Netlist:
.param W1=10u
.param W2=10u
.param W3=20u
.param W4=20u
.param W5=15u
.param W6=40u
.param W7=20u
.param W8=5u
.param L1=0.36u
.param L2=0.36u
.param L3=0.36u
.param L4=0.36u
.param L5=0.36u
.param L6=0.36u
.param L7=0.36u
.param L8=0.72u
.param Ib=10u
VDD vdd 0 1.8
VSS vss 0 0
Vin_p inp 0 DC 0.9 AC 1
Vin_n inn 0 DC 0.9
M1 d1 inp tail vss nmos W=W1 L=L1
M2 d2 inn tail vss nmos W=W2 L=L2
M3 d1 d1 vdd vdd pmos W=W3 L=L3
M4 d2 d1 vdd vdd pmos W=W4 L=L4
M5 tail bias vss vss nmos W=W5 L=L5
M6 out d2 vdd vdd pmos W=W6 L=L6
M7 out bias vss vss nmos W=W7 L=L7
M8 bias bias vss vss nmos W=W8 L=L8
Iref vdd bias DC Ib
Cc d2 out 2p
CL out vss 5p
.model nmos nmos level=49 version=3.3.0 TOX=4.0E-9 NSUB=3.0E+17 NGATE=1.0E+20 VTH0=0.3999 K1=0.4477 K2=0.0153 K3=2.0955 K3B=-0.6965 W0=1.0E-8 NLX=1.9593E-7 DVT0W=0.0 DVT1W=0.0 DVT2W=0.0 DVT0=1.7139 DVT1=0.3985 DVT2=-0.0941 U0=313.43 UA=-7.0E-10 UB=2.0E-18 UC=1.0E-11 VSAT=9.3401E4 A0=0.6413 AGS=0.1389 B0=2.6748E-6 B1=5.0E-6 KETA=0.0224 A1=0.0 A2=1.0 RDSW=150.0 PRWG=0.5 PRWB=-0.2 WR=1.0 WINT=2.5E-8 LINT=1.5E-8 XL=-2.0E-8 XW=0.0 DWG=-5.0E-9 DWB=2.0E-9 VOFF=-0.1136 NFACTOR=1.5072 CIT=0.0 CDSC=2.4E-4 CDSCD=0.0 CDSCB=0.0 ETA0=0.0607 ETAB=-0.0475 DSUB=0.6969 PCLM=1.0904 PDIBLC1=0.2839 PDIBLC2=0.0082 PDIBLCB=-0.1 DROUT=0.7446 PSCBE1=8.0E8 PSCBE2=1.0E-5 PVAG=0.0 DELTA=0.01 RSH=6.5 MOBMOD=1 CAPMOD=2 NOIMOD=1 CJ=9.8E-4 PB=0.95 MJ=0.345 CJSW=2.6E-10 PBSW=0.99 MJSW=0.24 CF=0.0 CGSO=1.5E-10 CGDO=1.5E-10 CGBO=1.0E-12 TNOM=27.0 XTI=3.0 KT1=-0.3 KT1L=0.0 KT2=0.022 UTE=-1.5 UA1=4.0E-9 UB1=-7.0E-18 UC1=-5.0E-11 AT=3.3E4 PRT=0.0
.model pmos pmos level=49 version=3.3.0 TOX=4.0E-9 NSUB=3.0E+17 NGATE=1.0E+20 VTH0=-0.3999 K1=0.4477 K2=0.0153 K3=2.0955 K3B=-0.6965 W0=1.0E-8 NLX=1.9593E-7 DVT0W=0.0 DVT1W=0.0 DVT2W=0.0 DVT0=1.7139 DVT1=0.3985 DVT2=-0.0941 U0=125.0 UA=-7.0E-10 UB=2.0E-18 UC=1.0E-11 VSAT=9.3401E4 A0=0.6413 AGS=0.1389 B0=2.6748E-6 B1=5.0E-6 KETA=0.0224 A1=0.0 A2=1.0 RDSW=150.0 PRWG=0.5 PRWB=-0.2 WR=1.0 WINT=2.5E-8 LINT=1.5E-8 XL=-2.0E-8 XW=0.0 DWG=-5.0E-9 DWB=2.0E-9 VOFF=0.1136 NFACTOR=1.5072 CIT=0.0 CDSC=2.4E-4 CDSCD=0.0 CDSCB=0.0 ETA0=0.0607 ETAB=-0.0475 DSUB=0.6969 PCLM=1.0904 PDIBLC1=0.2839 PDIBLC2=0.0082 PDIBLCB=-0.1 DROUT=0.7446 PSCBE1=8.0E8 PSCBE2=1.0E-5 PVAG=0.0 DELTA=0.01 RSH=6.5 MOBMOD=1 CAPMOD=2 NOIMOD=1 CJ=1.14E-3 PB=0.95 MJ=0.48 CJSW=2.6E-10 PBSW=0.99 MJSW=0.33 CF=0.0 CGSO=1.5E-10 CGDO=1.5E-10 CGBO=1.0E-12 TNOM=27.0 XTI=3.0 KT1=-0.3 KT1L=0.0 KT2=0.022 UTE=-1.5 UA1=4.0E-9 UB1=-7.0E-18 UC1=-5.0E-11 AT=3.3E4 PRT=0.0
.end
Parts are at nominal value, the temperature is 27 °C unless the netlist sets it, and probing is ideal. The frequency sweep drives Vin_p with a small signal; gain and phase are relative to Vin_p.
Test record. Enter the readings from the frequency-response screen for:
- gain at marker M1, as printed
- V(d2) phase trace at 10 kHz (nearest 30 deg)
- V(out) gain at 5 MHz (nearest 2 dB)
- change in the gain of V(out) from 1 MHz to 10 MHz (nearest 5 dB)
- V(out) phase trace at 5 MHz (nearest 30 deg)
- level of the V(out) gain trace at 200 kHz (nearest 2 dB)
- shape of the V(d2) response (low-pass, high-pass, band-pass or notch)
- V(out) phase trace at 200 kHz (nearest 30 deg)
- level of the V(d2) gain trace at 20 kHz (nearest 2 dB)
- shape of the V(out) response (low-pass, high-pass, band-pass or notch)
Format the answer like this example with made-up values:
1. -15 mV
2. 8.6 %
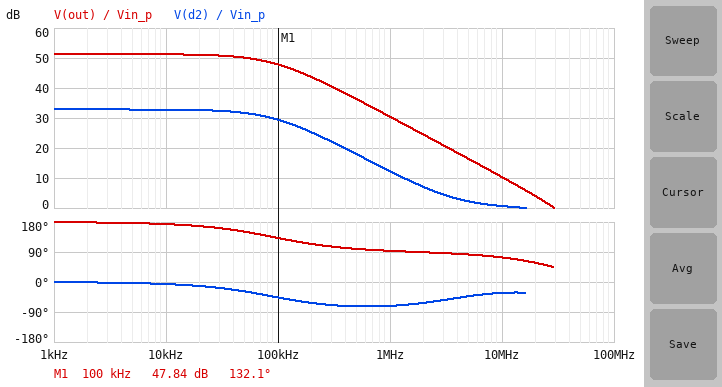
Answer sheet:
1. 47.84 dB
2. 0 deg
3. 16 dB
4. -20 dB
5. 90 deg
6. 44 dB
7. low-pass
8. 120 deg
9. 32 dB
10. low-pass
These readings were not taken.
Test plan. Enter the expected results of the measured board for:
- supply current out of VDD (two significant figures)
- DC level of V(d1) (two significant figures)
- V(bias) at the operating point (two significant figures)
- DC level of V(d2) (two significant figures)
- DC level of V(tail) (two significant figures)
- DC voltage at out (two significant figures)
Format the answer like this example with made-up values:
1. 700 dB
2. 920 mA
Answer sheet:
1. 130 µA
2. 1.0 V
3. 540 mV
4. 1.0 V
5. 320 mV
6. 110 mV
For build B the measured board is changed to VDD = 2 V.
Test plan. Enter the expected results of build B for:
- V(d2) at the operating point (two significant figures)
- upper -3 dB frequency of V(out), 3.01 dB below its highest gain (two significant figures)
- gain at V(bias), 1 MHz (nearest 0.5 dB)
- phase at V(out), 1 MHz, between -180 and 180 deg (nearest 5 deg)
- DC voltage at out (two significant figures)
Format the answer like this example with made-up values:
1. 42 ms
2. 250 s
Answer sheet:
1. 1.2 V
2. 65 kHz
3. -46.0 dB
4. 90 deg
5. 120 mV
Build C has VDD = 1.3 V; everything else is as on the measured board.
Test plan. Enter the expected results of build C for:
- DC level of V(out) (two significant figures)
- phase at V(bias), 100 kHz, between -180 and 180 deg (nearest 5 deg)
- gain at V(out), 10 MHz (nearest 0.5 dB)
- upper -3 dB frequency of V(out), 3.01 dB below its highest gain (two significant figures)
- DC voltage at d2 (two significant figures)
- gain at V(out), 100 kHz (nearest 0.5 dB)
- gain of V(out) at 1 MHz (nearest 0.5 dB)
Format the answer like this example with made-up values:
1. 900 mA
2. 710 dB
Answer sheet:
1. 86 mV
2. -110 deg
3. 9.0 dB
4. 260 kHz
5. 500 mV
6. 40.5 dB
7. 29.0 dB
